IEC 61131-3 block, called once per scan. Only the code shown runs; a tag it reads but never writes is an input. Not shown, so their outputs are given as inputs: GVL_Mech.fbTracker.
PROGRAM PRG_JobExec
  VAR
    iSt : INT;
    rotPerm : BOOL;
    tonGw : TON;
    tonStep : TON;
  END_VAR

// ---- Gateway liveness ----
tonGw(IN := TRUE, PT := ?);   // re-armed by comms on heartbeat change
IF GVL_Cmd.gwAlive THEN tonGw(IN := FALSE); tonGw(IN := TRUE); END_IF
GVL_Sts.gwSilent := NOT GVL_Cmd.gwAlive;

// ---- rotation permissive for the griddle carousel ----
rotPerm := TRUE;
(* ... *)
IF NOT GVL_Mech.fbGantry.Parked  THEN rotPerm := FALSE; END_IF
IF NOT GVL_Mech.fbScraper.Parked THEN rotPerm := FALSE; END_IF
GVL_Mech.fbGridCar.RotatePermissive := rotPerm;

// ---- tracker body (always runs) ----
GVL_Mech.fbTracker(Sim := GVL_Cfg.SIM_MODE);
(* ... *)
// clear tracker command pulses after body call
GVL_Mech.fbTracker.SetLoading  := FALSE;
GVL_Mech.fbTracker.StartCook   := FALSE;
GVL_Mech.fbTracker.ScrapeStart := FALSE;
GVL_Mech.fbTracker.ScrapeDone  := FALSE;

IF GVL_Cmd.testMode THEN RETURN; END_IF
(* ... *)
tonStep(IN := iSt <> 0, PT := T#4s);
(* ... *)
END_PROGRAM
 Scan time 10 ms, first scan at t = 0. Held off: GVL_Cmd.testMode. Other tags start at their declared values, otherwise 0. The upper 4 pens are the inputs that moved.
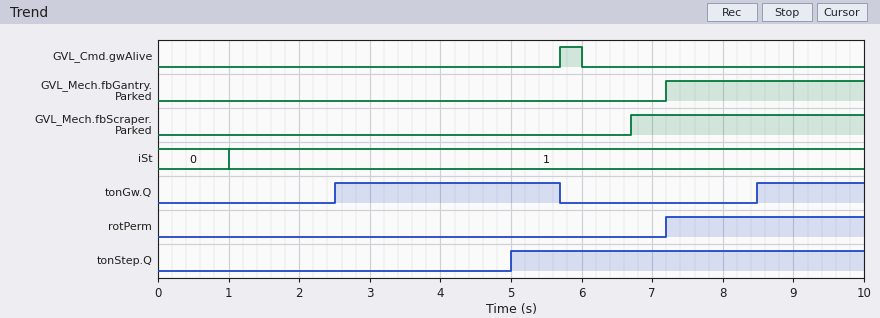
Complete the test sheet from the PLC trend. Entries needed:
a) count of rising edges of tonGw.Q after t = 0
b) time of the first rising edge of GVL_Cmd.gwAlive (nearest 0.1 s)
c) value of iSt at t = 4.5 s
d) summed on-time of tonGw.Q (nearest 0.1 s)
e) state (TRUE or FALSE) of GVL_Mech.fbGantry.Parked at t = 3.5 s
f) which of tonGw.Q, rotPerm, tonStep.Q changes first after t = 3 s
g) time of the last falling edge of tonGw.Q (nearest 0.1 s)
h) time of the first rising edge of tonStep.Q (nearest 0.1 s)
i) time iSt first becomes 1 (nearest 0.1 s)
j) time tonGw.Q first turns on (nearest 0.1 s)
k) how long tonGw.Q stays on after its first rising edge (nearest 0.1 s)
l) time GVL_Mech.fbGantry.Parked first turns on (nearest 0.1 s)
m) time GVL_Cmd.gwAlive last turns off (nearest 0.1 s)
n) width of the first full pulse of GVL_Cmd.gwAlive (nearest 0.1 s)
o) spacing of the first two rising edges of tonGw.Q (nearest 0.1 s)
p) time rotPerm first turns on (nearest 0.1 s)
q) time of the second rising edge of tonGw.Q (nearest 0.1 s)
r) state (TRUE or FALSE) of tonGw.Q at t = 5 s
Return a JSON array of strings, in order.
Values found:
["2", "5.7 s", "1", "4.7 s", "FALSE", "tonStep.Q", "5.7 s", "5.0 s", "1.0 s", "2.5 s", "3.2 s", "7.2 s", "6.0 s", "0.3 s", "6.0 s", "7.2 s", "8.5 s", "TRUE"]
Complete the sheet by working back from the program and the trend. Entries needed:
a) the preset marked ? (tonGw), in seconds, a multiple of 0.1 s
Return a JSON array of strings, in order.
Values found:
["2.5 s"]
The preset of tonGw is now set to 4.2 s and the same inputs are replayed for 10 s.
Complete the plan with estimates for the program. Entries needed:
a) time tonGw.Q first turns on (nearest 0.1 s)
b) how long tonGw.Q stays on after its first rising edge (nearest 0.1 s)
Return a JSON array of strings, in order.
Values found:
["4.2 s", "1.5 s"]
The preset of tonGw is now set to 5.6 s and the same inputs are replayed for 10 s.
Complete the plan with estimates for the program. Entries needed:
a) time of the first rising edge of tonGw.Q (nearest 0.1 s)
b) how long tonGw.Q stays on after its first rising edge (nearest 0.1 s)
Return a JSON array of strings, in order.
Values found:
["5.6 s", "0.1 s"]
